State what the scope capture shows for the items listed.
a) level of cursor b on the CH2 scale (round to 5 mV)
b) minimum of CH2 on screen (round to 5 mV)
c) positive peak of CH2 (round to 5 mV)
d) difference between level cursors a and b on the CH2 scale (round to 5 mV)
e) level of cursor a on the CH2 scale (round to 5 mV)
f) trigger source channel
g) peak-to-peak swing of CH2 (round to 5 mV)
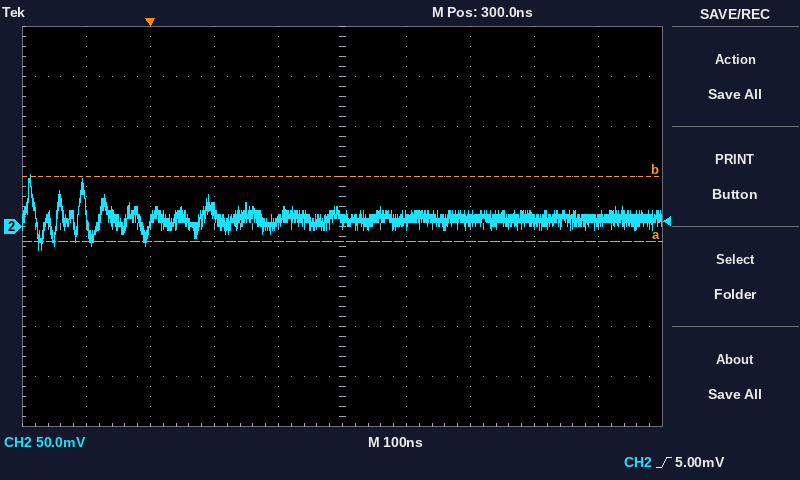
50 mV
-25 mV
50 mV
65 mV
-15 mV
CH2
75 mV
